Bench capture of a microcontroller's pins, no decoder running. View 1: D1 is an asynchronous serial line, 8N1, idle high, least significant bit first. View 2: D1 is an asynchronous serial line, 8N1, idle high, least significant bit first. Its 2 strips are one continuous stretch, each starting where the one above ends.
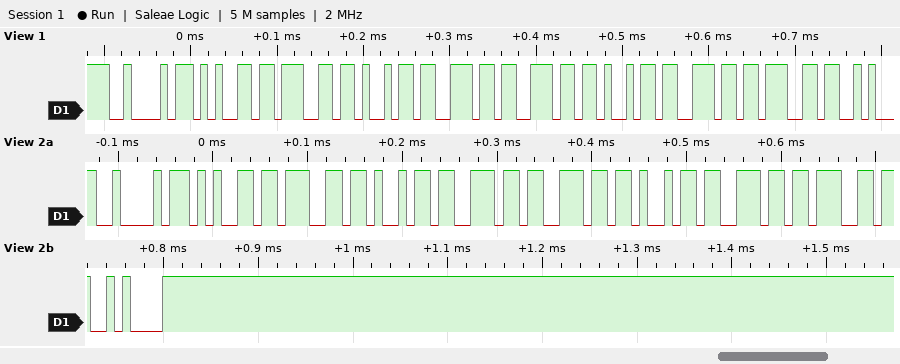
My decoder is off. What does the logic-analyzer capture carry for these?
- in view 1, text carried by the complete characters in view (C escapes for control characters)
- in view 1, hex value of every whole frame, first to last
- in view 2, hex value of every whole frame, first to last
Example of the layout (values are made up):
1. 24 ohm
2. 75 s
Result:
1. "Beginning"
2. 0x42 0x65 0x67 0x69 0x6E 0x6E 0x69 0x6E 0x67
3. 42 65 67 69 6E 6E 69 6E 67 0A
